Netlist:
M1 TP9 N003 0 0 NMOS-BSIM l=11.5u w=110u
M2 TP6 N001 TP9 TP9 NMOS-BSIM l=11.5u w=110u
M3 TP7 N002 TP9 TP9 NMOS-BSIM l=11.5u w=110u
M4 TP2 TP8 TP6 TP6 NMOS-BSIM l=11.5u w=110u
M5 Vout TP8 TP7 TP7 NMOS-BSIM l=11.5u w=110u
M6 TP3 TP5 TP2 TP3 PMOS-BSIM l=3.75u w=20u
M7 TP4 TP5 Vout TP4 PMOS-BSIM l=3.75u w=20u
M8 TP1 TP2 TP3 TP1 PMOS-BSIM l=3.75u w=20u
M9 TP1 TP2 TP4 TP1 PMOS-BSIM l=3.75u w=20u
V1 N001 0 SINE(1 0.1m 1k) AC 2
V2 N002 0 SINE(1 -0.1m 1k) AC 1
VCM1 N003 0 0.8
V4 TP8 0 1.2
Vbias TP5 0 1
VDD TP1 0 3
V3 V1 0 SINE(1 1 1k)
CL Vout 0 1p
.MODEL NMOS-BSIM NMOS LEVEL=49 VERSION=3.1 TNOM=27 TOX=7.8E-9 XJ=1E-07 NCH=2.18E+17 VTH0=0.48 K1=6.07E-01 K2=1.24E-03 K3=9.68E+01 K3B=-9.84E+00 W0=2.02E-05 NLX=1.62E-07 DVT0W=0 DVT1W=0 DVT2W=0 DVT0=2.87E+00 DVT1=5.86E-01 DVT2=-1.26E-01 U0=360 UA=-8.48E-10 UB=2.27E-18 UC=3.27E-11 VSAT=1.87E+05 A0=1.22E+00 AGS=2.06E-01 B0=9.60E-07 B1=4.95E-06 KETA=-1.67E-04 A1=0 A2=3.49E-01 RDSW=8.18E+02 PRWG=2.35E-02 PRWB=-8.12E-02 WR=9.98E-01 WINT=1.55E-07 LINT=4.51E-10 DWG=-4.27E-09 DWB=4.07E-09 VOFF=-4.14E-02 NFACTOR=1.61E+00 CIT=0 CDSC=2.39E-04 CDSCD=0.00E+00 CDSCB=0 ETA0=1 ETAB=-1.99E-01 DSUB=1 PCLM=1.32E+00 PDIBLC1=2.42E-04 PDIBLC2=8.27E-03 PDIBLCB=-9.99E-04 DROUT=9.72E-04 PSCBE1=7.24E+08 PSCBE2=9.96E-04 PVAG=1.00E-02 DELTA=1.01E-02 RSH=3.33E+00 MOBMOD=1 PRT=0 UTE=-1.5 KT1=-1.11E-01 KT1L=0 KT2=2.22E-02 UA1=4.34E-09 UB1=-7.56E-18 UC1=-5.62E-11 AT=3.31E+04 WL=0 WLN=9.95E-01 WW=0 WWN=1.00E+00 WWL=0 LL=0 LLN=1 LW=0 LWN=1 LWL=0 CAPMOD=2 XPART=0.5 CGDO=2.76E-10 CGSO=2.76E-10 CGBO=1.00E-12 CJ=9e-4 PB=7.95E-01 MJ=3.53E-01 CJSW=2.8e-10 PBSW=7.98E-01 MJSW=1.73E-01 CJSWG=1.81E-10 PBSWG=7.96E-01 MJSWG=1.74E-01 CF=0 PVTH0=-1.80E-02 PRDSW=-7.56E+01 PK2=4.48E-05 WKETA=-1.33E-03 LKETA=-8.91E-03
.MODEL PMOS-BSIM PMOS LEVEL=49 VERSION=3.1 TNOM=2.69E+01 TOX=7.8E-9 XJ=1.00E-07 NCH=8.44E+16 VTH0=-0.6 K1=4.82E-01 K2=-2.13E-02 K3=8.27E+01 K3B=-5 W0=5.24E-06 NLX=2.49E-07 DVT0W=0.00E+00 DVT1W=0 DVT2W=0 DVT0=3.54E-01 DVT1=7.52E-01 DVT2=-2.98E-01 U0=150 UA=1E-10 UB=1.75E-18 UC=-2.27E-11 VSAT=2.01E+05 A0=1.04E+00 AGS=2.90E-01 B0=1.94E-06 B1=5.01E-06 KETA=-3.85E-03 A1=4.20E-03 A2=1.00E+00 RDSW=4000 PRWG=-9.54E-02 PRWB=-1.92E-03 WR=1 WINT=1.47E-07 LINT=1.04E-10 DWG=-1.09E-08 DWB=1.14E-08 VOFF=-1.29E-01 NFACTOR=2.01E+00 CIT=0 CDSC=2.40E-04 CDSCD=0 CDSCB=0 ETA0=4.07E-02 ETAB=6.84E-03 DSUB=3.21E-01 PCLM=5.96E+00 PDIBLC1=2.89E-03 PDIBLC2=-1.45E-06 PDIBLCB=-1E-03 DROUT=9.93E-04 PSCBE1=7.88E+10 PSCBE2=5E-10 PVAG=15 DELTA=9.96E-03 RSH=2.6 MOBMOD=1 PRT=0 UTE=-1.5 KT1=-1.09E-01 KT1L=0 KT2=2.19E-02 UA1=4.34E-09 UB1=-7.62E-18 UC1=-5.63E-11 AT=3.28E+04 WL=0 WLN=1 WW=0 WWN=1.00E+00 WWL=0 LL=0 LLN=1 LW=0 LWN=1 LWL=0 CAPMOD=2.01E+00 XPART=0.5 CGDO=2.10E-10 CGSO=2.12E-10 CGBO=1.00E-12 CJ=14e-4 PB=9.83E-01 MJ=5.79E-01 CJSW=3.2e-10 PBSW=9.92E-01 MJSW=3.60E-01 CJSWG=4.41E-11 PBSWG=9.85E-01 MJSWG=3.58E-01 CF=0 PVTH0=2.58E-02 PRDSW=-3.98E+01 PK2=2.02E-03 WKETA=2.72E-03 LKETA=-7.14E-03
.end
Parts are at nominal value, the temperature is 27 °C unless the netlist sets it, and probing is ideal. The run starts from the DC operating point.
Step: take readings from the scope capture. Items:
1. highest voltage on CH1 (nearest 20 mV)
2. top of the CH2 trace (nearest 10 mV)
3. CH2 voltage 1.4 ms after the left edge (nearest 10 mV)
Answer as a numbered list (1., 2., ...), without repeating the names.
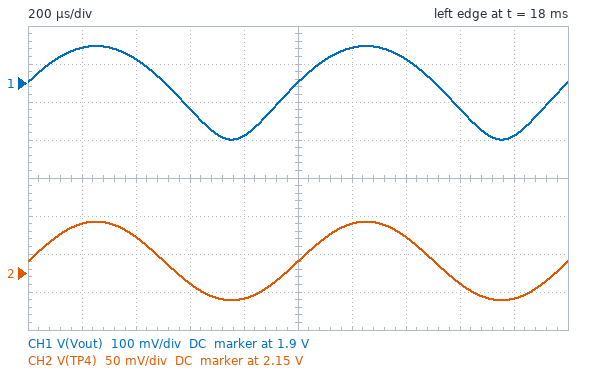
1. 2.00 V
2. 2.22 V
3. 2.20 V
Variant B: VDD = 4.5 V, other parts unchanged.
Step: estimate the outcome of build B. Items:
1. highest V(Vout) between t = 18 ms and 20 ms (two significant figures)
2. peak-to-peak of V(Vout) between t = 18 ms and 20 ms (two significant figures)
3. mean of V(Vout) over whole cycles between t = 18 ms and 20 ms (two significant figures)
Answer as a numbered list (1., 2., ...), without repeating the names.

1. 3.5 V
2. 130 mV
3. 3.4 V
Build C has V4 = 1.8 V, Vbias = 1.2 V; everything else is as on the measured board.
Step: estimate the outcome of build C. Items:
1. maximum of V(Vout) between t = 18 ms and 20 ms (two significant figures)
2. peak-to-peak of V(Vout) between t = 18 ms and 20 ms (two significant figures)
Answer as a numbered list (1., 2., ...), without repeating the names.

1. 2.1 V
2. 960 mV
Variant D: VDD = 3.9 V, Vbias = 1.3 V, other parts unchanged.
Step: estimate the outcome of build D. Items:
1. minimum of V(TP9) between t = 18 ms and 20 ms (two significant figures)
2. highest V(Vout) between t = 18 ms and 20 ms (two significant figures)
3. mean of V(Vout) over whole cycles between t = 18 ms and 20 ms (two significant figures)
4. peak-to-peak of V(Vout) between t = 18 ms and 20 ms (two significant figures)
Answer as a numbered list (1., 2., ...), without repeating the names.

1. 280 mV
2. 2.9 V
3. 2.8 V
4. 140 mV
